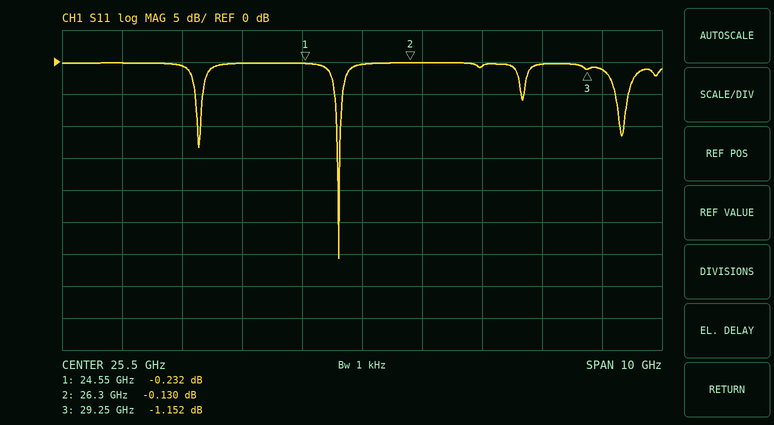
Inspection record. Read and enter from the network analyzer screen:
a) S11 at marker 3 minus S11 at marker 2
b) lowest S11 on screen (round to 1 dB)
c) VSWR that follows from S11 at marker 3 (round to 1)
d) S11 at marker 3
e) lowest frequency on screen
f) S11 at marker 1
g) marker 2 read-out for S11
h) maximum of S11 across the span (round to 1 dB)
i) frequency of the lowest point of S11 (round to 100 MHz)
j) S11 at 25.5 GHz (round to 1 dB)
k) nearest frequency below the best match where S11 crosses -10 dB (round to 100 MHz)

-1.022 dB
-31 dB
15
-1.152 dB
20.5 GHz
-0.232 dB
-0.130 dB
0 dB
25.1 GHz
0 dB
25.1 GHz
